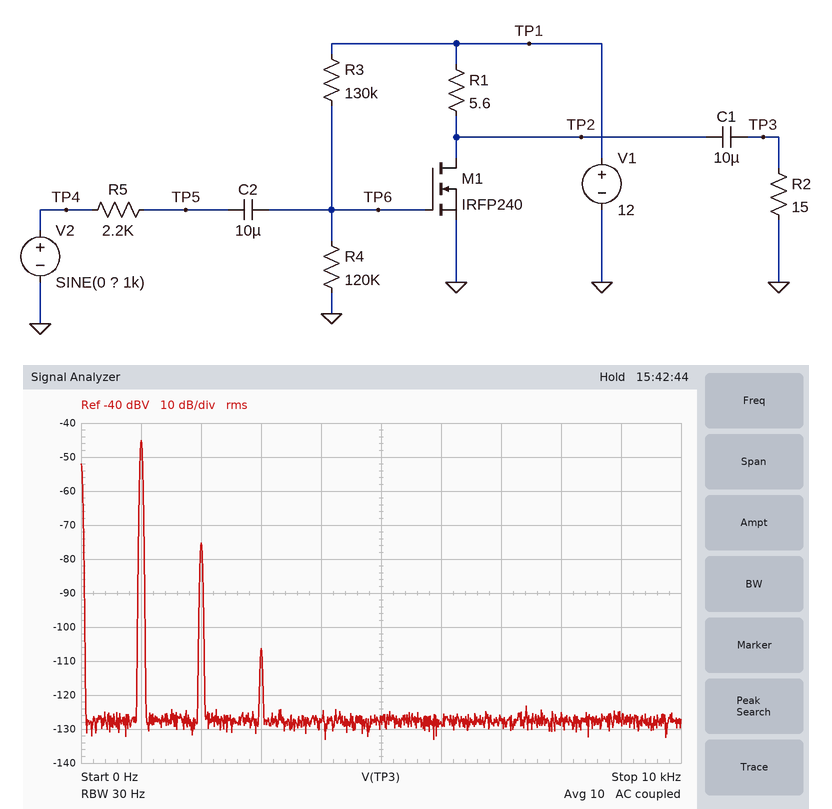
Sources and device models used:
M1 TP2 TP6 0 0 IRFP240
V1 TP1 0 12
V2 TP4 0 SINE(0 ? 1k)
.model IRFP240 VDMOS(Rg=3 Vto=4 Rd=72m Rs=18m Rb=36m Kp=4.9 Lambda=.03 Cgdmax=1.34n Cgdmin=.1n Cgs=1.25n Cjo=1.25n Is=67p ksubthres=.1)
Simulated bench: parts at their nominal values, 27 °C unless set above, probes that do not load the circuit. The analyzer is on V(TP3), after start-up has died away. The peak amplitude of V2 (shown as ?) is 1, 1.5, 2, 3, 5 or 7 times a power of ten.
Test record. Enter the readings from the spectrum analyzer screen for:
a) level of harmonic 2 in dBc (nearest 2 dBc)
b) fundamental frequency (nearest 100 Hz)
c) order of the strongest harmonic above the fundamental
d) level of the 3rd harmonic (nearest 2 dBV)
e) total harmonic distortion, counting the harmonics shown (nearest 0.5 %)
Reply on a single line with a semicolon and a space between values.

-30 dBc; 1.0 kHz; 2; -106 dBV; 3.0 %
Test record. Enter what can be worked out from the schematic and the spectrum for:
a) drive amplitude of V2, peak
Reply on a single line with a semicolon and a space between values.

70 mV
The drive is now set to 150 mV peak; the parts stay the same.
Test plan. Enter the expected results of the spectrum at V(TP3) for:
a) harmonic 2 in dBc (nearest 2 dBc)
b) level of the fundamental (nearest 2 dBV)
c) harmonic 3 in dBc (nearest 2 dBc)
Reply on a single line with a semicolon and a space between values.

-24 dBc; -38 dBV; -48 dBc
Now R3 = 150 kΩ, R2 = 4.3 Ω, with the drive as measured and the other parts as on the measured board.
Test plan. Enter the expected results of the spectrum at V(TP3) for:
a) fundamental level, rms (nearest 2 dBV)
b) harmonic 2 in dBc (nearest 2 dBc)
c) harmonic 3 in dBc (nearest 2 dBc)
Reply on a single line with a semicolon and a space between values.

-46 dBV; -22 dBc; -46 dBc
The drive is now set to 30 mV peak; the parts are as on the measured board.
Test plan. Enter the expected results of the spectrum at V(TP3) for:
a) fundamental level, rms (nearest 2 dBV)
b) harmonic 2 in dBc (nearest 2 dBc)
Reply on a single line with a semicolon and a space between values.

-52 dBV; -38 dBc
